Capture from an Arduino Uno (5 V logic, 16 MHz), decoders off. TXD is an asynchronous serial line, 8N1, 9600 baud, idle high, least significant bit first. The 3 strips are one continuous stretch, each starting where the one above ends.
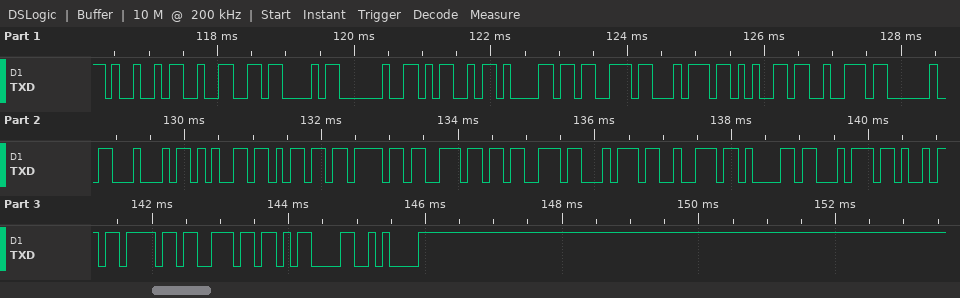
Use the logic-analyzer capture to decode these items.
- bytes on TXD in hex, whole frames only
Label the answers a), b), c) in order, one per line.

a) 49 32 43 20 4D 61 73 74 65 72 20 44 65 6D 6F 6E 73 74 72 61 74 69 6F 6E 0D 0A
